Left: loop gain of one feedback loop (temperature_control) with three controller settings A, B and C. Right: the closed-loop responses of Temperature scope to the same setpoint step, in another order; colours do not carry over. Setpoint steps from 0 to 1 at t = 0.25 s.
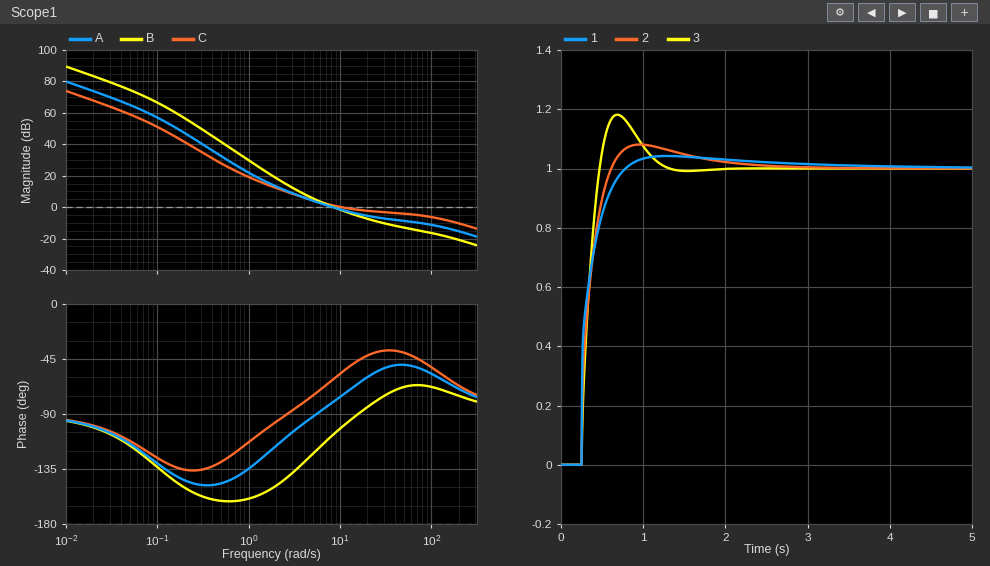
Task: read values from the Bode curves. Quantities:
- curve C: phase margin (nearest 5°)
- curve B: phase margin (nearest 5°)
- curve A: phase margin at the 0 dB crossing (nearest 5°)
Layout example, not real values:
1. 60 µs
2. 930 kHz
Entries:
1. 125°
2. 75°
3. 100°
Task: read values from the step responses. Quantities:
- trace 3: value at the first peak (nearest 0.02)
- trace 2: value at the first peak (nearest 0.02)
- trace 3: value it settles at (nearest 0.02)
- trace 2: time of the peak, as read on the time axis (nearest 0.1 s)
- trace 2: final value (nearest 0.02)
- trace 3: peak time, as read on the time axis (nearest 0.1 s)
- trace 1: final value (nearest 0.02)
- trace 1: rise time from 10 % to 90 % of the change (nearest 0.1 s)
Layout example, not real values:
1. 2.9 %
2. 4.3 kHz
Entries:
1. 1.18
2. 1.08
3. 1.00
4. 1.0 s
5. 1.00
6. 0.7 s
7. 1.00
8. 0.3 s
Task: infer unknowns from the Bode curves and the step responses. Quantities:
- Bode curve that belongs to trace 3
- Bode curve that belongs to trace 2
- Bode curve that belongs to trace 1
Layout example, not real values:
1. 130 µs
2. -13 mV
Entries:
1. B
2. A
3. C
